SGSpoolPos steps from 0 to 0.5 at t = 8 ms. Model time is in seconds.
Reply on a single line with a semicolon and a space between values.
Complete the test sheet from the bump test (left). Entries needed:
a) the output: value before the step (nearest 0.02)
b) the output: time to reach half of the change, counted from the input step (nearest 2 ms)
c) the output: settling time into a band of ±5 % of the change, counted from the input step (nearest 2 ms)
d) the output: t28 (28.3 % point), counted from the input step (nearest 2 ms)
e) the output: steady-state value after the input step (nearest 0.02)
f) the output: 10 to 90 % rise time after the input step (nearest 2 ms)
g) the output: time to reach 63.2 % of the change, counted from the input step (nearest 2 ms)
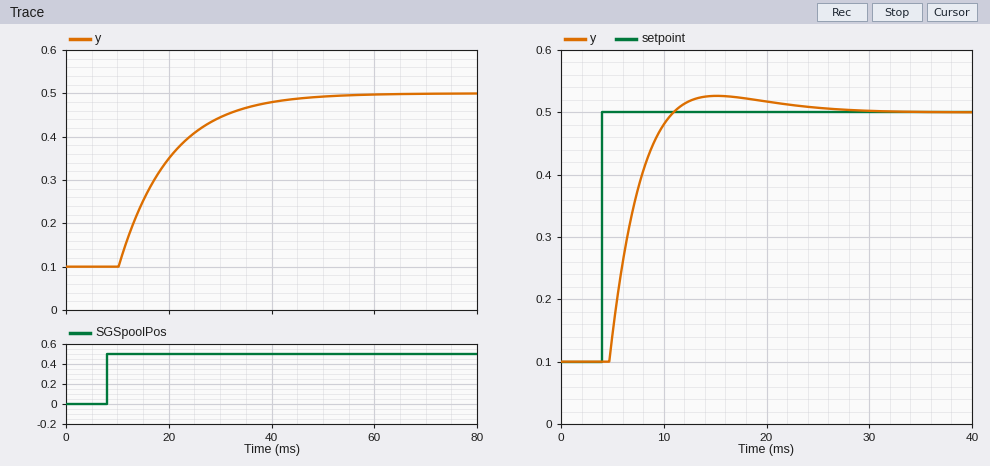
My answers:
0.10; 10 ms; 32 ms; 6 ms; 0.50; 22 ms; 12 ms
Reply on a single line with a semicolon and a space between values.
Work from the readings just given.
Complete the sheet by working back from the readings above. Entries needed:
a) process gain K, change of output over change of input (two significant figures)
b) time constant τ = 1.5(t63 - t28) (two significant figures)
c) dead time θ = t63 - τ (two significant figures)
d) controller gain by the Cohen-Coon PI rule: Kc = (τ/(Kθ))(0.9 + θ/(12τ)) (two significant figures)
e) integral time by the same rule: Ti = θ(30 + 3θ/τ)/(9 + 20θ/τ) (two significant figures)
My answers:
0.80; 9.0 ms; 3.0 ms; 3.5; 5.9 ms
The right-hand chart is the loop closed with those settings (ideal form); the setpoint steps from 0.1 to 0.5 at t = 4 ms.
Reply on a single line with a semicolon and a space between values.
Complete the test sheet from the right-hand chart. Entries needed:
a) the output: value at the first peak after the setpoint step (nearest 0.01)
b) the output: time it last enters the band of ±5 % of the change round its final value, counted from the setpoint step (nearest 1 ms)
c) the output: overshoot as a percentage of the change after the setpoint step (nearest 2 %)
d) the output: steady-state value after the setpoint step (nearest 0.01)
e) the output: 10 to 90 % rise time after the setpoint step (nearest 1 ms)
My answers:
0.53; 15 ms; 6 %; 0.50; 4 ms
